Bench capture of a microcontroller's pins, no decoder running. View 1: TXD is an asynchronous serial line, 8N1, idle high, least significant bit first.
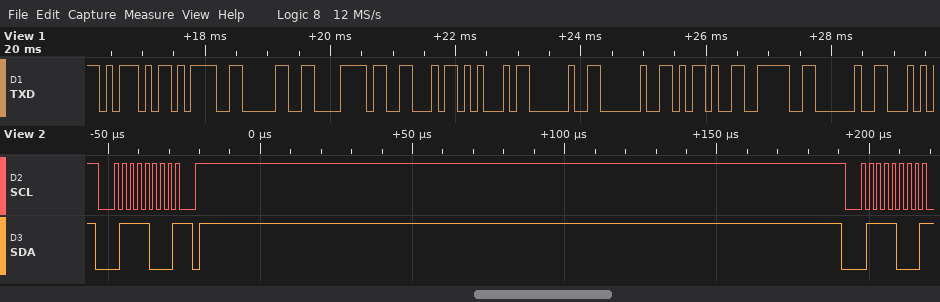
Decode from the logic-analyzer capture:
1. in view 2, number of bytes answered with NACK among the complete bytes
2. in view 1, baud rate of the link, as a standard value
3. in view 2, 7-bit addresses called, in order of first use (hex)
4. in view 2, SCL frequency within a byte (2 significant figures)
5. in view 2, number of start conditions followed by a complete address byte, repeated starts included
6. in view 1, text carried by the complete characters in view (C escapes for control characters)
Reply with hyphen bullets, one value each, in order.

- 2
- 9600 baud
- 0x3C
- 400 kHz
- 2
- "]=0xFE  -> "
